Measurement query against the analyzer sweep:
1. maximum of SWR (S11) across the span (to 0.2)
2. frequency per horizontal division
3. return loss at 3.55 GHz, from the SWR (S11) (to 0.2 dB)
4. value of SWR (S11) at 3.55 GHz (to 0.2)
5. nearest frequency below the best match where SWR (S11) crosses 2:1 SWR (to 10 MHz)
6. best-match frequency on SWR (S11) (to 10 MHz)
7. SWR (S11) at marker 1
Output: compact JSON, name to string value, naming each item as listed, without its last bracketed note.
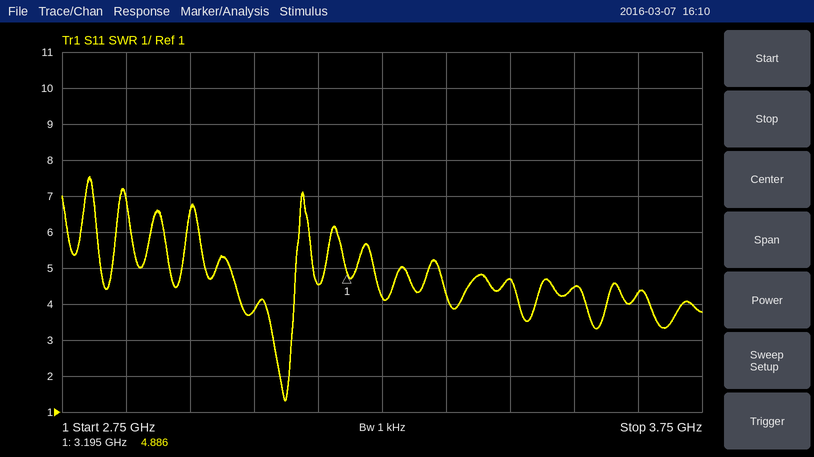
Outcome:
{"maximum of SWR (S11) across the span": "7.6", "frequency per horizontal division": "100 MHz", "return loss at 3.55 GHz, from the SWR (S11)": "4.0 dB", "value of SWR (S11) at 3.55 GHz": "4.4", "nearest frequency below the best match where SWR (S11) crosses 2:1 SWR": "3.09 GHz", "best-match frequency on SWR (S11)": "3.10 GHz", "SWR (S11) at marker 1": "4.886"}
